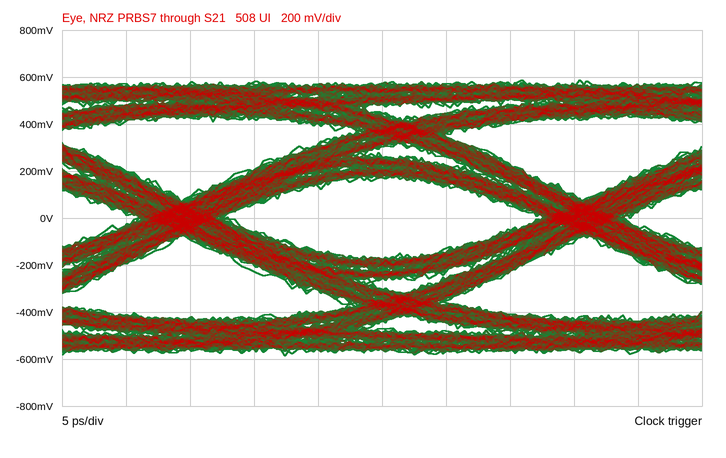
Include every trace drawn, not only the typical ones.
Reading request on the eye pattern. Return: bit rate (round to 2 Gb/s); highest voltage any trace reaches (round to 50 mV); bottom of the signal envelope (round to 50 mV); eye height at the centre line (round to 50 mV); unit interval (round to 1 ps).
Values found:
32 Gb/s
600 mV
-600 mV
350 mV
31 ps
